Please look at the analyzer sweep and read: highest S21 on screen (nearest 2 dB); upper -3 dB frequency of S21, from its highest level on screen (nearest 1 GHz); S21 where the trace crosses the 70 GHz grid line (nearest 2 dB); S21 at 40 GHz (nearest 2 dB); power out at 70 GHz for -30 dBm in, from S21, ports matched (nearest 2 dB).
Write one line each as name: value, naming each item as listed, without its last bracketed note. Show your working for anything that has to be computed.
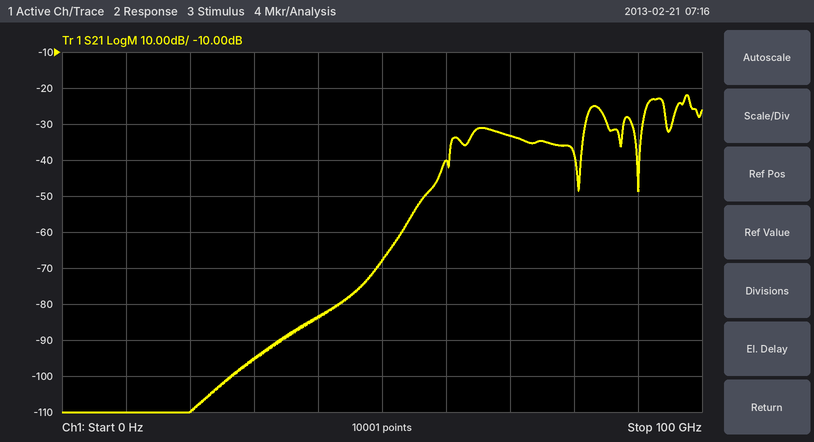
highest S21 on screen: -22 dB
upper -3 dB frequency of S21, from its highest level on screen: 98 GHz
S21 where the trace crosses the 70 GHz grid line: -34 dB
S21 at 40 GHz: -84 dB
power out at 70 GHz for -30 dBm in, from S21, ports matched: -30 dBm + (-34 dB) = -64 dBm
